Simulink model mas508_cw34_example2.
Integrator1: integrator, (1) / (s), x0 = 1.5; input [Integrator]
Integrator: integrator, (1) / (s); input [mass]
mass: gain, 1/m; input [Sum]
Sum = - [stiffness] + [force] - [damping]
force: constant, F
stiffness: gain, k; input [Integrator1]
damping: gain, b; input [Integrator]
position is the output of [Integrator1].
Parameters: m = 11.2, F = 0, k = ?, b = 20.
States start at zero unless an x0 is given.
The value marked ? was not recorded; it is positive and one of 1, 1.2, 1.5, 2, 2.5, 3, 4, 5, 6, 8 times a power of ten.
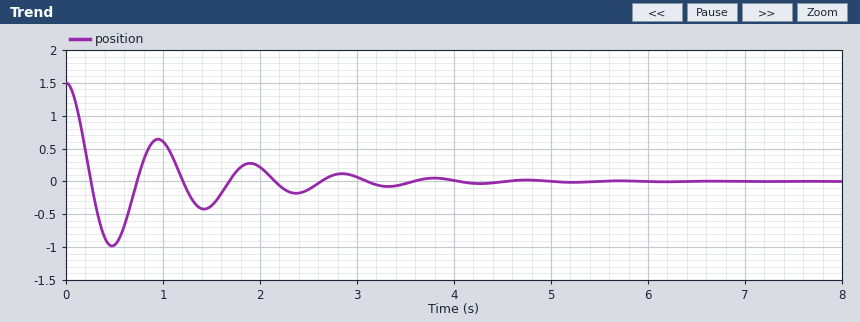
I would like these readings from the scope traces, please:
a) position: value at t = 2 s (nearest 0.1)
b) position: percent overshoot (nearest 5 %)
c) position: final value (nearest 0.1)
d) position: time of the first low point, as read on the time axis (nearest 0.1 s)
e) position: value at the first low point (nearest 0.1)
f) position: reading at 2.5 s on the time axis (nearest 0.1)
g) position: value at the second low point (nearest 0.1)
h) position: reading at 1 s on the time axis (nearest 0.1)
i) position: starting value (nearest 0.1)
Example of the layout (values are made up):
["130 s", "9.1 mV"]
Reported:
["0.2", "65 %", "0.0", "0.5 s", "-1.0", "-0.1", "-0.4", "0.6", "1.5"]
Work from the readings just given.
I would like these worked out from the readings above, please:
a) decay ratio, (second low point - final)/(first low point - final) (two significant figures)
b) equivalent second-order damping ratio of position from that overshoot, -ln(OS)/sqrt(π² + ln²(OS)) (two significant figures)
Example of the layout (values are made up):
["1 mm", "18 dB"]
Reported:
["0.40", "0.14"]
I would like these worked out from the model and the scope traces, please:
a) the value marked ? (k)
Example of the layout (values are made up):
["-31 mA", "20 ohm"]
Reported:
["500"]
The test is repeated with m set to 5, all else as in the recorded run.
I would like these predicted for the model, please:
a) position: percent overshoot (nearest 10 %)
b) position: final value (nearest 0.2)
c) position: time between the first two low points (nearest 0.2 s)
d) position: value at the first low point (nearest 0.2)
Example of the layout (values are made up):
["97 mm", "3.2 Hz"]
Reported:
["50 %", "0.0", "0.6 s", "-0.8"]
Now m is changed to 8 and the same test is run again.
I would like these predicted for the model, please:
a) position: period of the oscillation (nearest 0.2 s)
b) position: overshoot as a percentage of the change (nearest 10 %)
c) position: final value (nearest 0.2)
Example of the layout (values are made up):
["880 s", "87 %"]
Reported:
["0.8 s", "60 %", "0.0"]
